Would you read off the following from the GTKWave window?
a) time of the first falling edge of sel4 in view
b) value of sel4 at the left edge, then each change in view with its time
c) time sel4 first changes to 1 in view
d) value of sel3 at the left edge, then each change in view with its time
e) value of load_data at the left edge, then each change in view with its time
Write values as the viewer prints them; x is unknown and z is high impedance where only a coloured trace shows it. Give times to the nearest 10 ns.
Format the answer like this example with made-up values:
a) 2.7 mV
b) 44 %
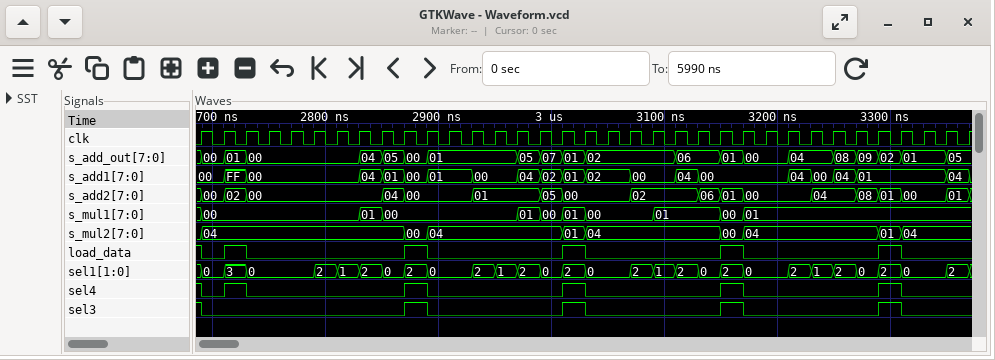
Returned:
a) 2690 ns
b) 1, 0 at 2690 ns, 1 at 2710 ns, 0 at 2730 ns, 1 at 2870 ns, 0 at 2890 ns, 1 at 3010 ns, 0 at 3030 ns, 1 at 3150 ns, 0 at 3170 ns, 1 at 3290 ns, 0 at 3310 ns
c) 2710 ns
d) 1, 0 at 2690 ns, 1 at 2870 ns, 0 at 2890 ns, 1 at 3010 ns, 0 at 3030 ns, 1 at 3150 ns, 0 at 3170 ns, 1 at 3290 ns, 0 at 3310 ns
e) 1, 0 at 2690 ns, 1 at 2710 ns, 0 at 2730 ns, 1 at 2870 ns, 0 at 2890 ns, 1 at 3010 ns, 0 at 3030 ns, 1 at 3150 ns, 0 at 3170 ns, 1 at 3290 ns, 0 at 3310 ns
